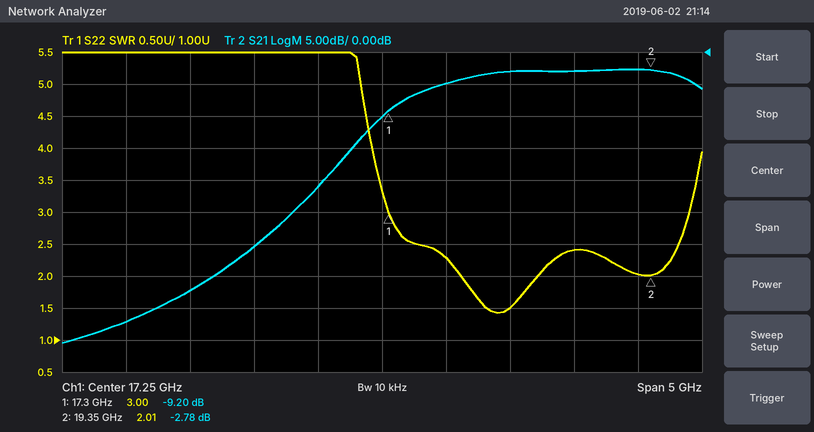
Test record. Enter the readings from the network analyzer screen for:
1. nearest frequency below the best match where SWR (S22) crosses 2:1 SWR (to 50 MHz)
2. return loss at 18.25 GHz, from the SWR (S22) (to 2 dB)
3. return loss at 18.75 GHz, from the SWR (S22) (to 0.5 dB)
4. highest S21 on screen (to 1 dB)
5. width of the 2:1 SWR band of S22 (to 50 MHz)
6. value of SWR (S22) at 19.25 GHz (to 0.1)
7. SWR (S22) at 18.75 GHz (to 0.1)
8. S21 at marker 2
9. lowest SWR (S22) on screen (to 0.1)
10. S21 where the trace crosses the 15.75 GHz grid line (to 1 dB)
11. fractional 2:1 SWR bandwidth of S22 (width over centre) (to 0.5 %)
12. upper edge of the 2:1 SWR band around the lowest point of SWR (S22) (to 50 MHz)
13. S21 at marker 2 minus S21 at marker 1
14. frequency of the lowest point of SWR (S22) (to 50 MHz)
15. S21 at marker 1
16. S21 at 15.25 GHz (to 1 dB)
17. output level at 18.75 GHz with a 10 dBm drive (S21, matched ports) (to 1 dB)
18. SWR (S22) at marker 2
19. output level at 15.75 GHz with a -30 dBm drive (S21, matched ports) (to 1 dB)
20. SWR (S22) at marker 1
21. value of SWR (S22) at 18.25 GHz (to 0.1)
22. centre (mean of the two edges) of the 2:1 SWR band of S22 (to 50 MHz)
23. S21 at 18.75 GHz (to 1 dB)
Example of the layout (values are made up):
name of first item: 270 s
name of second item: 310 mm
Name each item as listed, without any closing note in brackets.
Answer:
nearest frequency below the best match where SWR (S22) crosses 2:1 SWR: 17.85 GHz
return loss at 18.25 GHz, from the SWR (S22): 14 dB
return loss at 18.75 GHz, from the SWR (S22): 7.5 dB
highest S21 on screen: -3 dB
width of the 2:1 SWR band of S22: 600 MHz
value of SWR (S22) at 19.25 GHz: 2.0
SWR (S22) at 18.75 GHz: 2.4
S21 at marker 2: -2.78 dB
lowest SWR (S22) on screen: 1.4
S21 where the trace crosses the 15.75 GHz grid line: -37 dB
fractional 2:1 SWR bandwidth of S22 (width over centre): 3.5 %
upper edge of the 2:1 SWR band around the lowest point of SWR (S22): 18.45 GHz
S21 at marker 2 minus S21 at marker 1: 6.42 dB
frequency of the lowest point of SWR (S22): 18.15 GHz
S21 at marker 1: -9.20 dB
S21 at 15.25 GHz: -42 dB
output level at 18.75 GHz with a 10 dBm drive (S21, matched ports): 7 dBm
SWR (S22) at marker 2: 2.01
output level at 15.75 GHz with a -30 dBm drive (S21, matched ports): -67 dBm
SWR (S22) at marker 1: 3.00
value of SWR (S22) at 18.25 GHz: 1.5
centre (mean of the two edges) of the 2:1 SWR band of S22: 18.15 GHz
S21 at 18.75 GHz: -3 dB
